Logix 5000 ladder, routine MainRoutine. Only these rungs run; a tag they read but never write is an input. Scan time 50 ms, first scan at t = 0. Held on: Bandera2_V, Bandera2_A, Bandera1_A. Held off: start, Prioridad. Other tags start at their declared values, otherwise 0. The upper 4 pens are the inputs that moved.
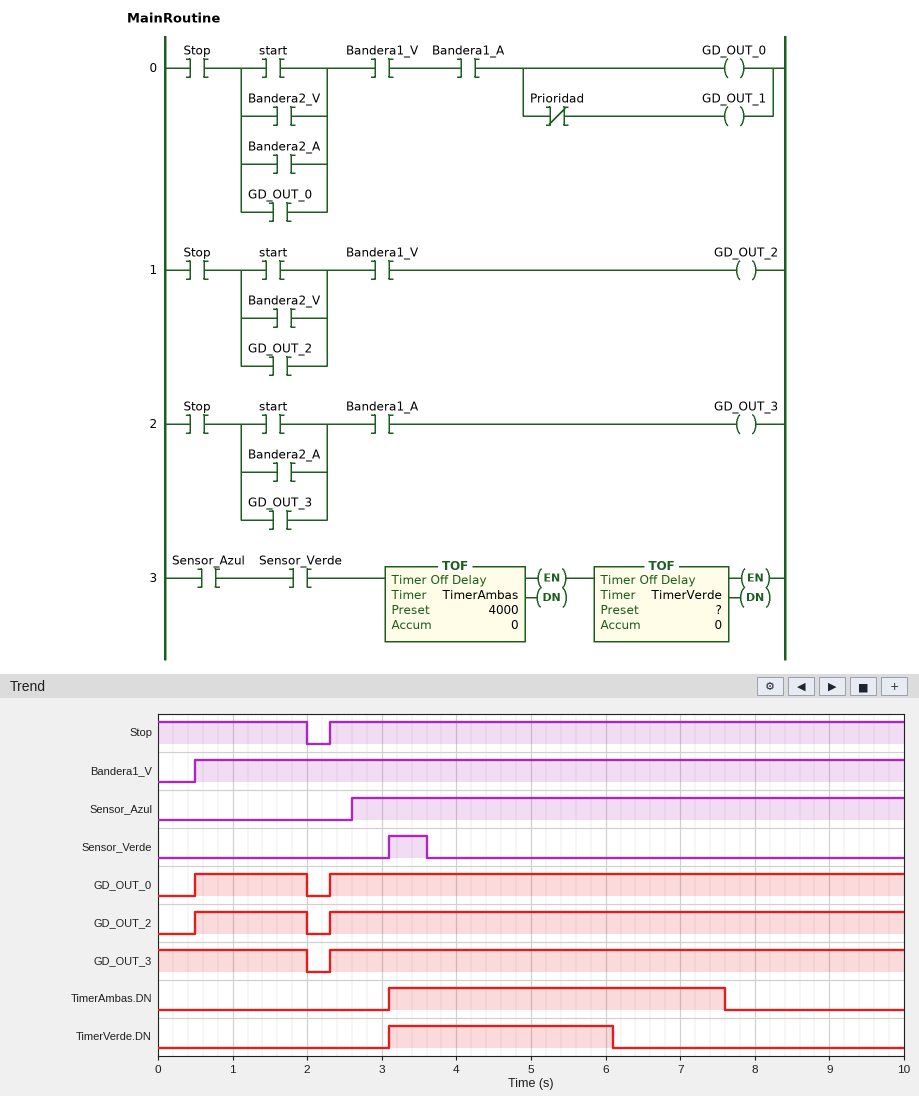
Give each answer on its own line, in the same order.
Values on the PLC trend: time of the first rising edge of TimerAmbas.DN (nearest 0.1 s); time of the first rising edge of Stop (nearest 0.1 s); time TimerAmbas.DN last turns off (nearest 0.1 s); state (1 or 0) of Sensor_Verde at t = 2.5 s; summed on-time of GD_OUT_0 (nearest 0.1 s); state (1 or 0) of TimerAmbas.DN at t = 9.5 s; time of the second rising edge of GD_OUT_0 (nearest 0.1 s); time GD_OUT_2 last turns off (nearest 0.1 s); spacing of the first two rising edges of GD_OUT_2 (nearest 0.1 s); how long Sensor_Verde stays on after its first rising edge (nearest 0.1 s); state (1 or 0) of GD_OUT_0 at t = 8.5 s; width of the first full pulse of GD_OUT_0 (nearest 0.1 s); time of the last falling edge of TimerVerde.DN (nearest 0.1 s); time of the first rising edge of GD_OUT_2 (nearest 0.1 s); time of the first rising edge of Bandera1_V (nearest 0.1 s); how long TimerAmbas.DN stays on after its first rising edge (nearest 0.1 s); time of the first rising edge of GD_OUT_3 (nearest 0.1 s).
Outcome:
3.1 s
2.3 s
7.6 s
0
9.2 s
0
2.3 s
2.0 s
1.8 s
0.5 s
1
1.5 s
6.1 s
0.5 s
0.5 s
4.5 s
2.3 s
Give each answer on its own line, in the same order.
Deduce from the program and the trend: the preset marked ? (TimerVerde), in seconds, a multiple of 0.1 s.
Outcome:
2.5 s
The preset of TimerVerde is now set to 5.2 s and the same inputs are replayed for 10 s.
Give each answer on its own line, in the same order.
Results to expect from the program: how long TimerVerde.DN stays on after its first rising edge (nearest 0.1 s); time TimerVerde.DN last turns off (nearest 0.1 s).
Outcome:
5.7 s
8.8 s
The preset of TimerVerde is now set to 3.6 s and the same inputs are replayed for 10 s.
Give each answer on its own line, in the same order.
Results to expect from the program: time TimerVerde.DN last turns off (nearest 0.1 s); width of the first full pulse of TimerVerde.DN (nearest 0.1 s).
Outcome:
7.2 s
4.1 s
